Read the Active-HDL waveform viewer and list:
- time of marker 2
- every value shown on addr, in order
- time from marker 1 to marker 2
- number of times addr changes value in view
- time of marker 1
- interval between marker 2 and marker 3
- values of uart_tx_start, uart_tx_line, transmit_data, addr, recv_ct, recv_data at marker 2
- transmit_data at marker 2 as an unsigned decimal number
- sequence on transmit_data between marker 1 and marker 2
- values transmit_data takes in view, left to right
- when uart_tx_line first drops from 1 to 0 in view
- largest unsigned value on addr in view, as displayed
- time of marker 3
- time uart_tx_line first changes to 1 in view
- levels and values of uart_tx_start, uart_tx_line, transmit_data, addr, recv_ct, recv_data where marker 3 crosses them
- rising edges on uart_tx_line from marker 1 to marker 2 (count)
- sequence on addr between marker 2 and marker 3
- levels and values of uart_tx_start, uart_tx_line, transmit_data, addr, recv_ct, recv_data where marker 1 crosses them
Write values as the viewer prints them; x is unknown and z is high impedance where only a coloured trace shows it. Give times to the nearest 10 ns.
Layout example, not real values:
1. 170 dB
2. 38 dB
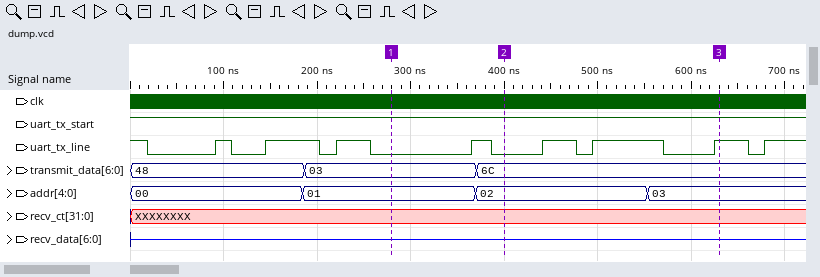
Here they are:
1. 400 ns
2. 00, 01, 02, 03
3. 120 ns
4. 3
5. 280 ns
6. 230 ns
7. uart_tx_start=1, uart_tx_line=0, transmit_data=6C, addr=02, recv_ct=XXXXXXXX, recv_data=z
8. 108
9. 03, 6C
10. 48, 03, 6C
11. 20 ns
12. 03
13. 630 ns
14. 90 ns
15. uart_tx_start=1, uart_tx_line=1, transmit_data=6C, addr=03, recv_ct=XXXXXXXX, recv_data=z
16. 1
17. 02, 03
18. uart_tx_start=1, uart_tx_line=0, transmit_data=03, addr=01, recv_ct=XXXXXXXX, recv_data=z
